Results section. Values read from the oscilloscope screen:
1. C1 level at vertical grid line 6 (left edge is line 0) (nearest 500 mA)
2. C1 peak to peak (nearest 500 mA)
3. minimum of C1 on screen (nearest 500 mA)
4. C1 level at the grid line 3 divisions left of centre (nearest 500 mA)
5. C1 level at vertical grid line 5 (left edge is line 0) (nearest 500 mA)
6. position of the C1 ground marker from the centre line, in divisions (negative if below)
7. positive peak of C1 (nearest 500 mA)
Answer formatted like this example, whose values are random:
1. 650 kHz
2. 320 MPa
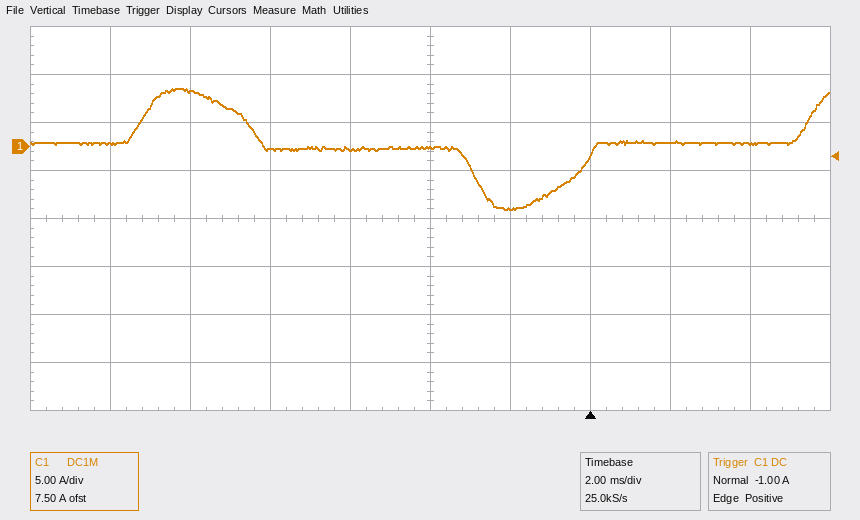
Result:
1. -6.5 A
2. 12.5 A
3. -6.5 A
4. 6.0 A
5. 0.0 A
6. +1.5 div
7. 6.0 A
